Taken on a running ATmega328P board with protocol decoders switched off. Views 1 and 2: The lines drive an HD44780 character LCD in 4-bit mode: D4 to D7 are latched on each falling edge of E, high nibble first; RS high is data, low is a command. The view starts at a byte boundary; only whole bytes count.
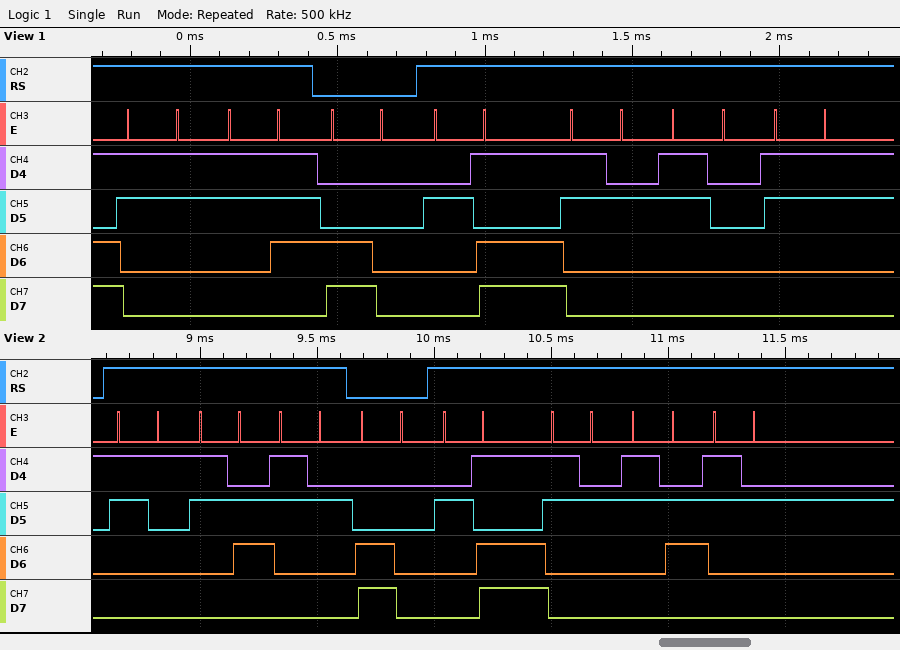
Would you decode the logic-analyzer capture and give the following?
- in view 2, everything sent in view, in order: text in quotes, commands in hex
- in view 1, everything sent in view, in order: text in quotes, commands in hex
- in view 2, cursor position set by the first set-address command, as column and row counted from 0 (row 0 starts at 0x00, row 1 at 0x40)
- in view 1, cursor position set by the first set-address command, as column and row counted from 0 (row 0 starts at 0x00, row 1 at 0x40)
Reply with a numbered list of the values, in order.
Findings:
1. "162" 0xC0 "-262"
2. "37" 0xC0 "-203"
3. column 0, row 1
4. column 0, row 1
